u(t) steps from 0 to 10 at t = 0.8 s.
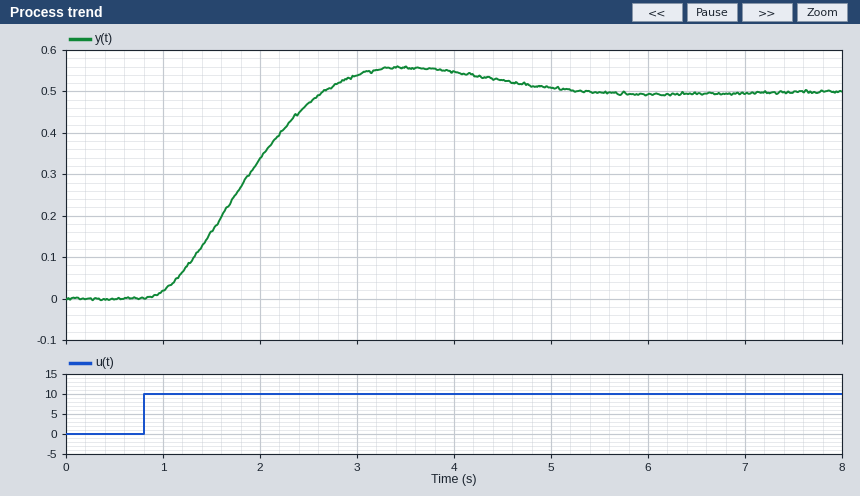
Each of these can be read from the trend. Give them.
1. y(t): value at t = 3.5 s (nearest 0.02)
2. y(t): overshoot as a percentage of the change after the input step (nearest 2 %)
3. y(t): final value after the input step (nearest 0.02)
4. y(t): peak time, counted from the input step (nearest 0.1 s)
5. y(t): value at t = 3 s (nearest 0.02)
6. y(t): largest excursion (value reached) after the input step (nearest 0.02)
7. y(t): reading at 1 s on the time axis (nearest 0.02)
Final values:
0.56
12 %
0.50
2.7 s
0.54
0.56
0.02
